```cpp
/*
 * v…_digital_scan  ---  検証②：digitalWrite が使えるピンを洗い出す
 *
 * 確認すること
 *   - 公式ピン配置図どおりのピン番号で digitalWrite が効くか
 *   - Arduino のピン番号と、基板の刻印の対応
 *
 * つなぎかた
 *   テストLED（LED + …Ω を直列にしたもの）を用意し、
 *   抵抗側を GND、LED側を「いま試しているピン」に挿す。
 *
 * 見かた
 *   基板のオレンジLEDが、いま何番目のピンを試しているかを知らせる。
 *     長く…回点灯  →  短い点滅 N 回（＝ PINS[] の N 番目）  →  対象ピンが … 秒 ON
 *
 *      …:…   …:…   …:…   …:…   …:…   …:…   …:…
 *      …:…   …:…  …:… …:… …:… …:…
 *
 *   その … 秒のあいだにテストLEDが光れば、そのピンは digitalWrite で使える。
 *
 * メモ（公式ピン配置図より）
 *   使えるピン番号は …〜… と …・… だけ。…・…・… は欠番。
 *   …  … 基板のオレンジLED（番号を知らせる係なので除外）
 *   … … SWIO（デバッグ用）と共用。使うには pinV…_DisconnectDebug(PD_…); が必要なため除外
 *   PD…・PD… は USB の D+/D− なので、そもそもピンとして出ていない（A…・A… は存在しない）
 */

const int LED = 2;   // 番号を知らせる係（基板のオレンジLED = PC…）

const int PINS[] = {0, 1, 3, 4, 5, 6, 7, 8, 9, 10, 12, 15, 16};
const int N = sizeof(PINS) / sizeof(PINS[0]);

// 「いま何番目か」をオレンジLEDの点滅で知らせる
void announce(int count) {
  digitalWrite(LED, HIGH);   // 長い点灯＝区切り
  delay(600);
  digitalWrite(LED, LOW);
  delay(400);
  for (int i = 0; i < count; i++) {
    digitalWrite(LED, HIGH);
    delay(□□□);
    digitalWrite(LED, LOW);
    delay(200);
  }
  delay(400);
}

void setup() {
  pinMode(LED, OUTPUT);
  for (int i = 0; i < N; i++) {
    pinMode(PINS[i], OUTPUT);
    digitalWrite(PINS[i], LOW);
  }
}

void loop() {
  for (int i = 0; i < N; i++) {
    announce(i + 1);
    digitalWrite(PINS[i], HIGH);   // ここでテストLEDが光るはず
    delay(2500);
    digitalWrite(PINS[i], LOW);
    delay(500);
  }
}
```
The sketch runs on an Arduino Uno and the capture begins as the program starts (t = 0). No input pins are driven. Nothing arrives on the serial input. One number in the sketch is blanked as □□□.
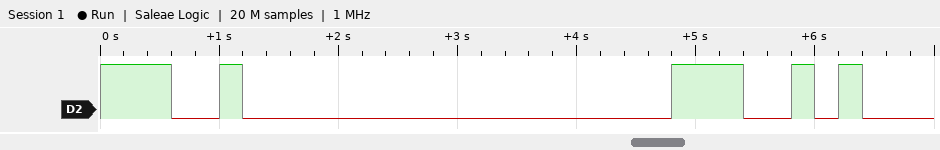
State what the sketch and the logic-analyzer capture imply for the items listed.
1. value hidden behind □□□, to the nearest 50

200
